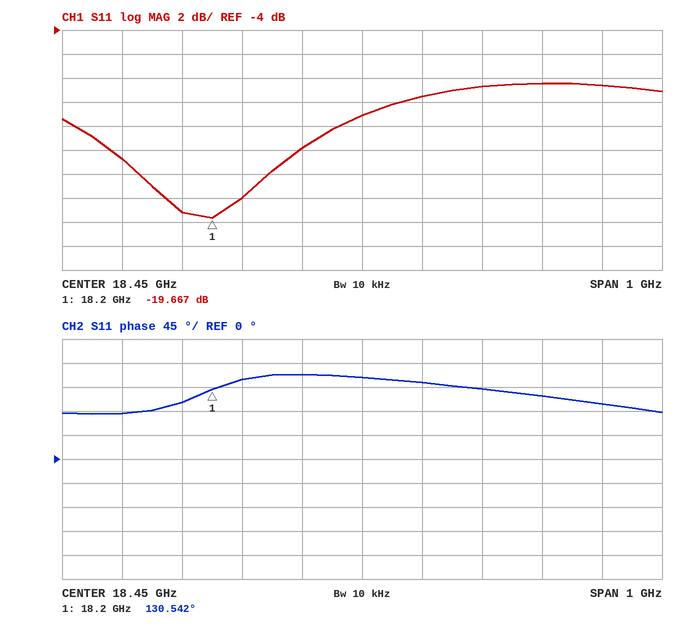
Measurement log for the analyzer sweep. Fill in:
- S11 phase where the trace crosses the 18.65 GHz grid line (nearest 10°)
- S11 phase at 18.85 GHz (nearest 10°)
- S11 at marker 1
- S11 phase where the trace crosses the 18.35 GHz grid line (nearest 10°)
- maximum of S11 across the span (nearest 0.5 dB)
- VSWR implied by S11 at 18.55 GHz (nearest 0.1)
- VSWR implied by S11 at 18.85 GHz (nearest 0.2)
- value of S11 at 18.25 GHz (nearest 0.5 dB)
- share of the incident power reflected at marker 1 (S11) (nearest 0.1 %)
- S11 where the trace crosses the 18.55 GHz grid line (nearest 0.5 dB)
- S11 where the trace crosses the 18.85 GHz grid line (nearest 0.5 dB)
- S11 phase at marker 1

130°
100°
-19.667 dB
160°
-8.5 dB
2.0
2.2
-18.0 dB
1.1 %
-9.5 dB
-8.5 dB
130.542°
